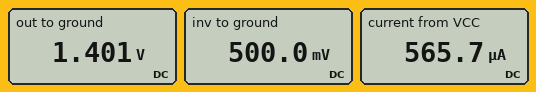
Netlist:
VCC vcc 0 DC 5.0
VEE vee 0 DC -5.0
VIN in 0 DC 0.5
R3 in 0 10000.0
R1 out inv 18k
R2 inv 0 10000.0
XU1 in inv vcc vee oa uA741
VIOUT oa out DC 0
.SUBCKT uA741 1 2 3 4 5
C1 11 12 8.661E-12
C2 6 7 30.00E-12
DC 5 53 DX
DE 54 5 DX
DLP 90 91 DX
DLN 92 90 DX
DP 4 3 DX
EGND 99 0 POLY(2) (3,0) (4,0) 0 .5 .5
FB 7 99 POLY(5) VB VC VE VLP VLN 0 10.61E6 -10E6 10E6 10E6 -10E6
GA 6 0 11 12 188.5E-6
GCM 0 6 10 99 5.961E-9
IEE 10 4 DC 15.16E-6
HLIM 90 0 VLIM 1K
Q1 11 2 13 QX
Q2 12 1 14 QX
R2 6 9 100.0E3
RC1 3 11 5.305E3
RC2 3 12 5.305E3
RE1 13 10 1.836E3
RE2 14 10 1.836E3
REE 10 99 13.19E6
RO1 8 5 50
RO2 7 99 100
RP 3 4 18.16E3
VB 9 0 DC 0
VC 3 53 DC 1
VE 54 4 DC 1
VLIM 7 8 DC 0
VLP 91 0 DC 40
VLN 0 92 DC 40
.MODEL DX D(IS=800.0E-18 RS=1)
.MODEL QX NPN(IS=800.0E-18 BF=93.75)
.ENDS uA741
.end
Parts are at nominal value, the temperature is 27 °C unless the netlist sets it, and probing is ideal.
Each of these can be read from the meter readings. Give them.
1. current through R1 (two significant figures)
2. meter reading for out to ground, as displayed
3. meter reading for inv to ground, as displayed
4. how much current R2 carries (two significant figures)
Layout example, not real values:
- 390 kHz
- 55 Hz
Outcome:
- 50 µA
- 1.401 V
- 500.0 mV
- 50 µA
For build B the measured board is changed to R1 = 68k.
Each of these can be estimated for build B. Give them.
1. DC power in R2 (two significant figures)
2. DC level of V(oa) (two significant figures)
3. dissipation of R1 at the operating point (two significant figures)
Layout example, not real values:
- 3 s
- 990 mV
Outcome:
- 25 µW
- 3.9 V
- 170 µW
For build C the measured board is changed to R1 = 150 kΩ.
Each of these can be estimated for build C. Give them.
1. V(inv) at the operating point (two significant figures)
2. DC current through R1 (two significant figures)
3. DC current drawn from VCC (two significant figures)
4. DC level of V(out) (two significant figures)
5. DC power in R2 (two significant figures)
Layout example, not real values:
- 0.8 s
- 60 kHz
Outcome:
- 290 mV
- 29 µA
- 550 µA
- 4.6 V
- 8.3 µW
